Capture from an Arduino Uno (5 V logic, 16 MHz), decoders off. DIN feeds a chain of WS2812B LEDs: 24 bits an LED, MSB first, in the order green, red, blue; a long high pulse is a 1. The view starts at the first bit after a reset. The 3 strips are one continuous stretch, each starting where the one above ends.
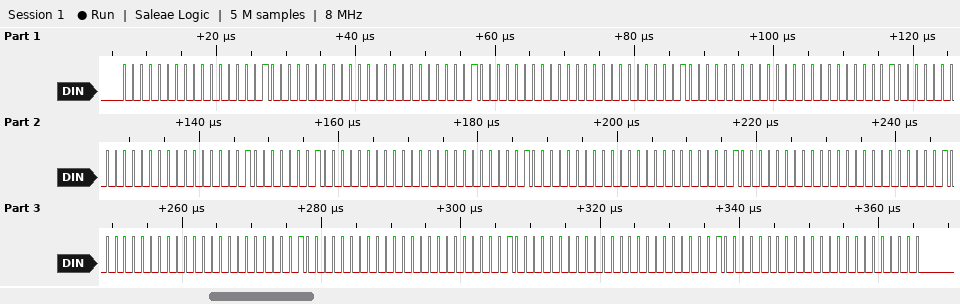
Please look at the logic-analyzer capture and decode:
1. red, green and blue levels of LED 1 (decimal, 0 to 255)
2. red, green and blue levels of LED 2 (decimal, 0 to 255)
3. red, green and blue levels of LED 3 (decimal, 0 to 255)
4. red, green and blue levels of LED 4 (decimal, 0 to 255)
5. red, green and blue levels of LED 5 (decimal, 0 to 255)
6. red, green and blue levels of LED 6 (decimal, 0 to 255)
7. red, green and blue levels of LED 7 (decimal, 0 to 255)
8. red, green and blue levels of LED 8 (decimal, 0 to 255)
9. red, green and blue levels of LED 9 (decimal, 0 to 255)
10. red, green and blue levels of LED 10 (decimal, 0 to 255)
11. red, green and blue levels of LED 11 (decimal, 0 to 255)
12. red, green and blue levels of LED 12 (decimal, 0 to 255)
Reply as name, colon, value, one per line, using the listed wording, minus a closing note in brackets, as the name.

red, green and blue levels of LED 1: 0, 0, 128
red, green and blue levels of LED 2: 0, 0, 128
red, green and blue levels of LED 3: 0, 0, 128
red, green and blue levels of LED 4: 0, 0, 128
red, green and blue levels of LED 5: 0, 0, 128
red, green and blue levels of LED 6: 0, 128, 0
red, green and blue levels of LED 7: 0, 128, 0
red, green and blue levels of LED 8: 0, 128, 0
red, green and blue levels of LED 9: 0, 128, 0
red, green and blue levels of LED 10: 0, 128, 0
red, green and blue levels of LED 11: 0, 128, 0
red, green and blue levels of LED 12: 0, 128, 0
